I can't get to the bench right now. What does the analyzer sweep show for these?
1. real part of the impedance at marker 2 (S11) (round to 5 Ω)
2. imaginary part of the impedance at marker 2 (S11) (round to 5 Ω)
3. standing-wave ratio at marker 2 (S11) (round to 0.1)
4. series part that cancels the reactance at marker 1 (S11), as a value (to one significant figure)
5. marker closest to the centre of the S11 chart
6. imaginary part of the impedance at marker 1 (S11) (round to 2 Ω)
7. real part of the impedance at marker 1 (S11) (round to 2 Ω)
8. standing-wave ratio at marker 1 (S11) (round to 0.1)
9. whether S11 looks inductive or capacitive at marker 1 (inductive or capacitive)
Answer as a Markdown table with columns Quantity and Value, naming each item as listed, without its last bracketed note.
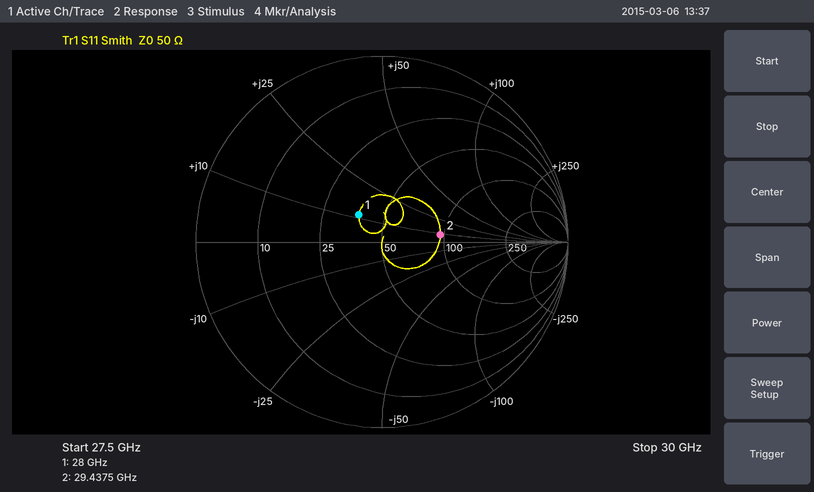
| Quantity | Value |
|---|---|
| real part of the impedance at marker 2 (S11) | 95 Ω |
| imaginary part of the impedance at marker 2 (S11) | +10 Ω |
| standing-wave ratio at marker 2 (S11) | 1.9 |
| series part that cancels the reactance at marker 1 (S11), as a value | 500 fF |
| marker closest to the centre of the S11 chart | marker 1 |
| imaginary part of the impedance at marker 1 (S11) | +12 Ω |
| real part of the impedance at marker 1 (S11) | 38 Ω |
| standing-wave ratio at marker 1 (S11) | 1.5 |
| whether S11 looks inductive or capacitive at marker 1 | inductive |
